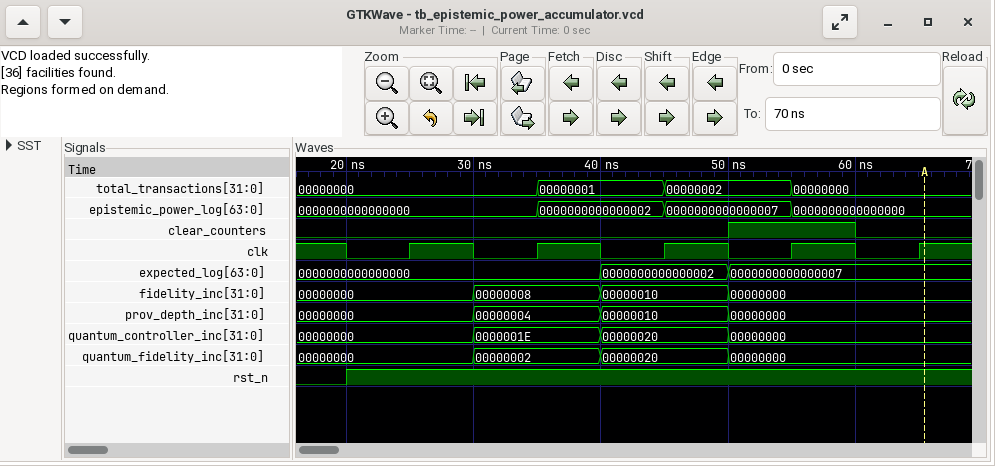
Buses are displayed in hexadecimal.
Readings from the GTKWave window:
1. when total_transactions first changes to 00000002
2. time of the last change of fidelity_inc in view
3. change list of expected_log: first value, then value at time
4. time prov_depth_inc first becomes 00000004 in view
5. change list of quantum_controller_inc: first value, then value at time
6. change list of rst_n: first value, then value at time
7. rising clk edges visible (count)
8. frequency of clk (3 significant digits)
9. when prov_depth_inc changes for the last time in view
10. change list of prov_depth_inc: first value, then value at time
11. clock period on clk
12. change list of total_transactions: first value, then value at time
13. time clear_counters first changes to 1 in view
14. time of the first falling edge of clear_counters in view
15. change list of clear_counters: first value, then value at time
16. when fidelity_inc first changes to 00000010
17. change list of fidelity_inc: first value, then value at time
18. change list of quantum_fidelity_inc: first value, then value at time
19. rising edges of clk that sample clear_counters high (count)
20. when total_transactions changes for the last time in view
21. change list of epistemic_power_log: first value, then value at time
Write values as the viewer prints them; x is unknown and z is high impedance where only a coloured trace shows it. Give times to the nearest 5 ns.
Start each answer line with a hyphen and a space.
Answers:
- 45 ns
- 50 ns
- 0000000000000000, 0000000000000002 at 40 ns, 0000000000000007 at 50 ns
- 30 ns
- 00000000, 0000001E at 30 ns, 00000020 at 40 ns, 00000000 at 50 ns
- 0, 1 at 20 ns
- 5
- 100 MHz
- 50 ns
- 00000000, 00000004 at 30 ns, 00000010 at 40 ns, 00000000 at 50 ns
- 10 ns
- 00000000, 00000001 at 35 ns, 00000002 at 45 ns, 00000000 at 55 ns
- 50 ns
- 60 ns
- 0, 1 at 50 ns, 0 at 60 ns
- 40 ns
- 00000000, 00000008 at 30 ns, 00000010 at 40 ns, 00000000 at 50 ns
- 00000000, 00000002 at 30 ns, 00000020 at 40 ns, 00000000 at 50 ns
- 1
- 55 ns
- 0000000000000000, 0000000000000002 at 35 ns, 0000000000000007 at 45 ns, 0000000000000000 at 55 ns
